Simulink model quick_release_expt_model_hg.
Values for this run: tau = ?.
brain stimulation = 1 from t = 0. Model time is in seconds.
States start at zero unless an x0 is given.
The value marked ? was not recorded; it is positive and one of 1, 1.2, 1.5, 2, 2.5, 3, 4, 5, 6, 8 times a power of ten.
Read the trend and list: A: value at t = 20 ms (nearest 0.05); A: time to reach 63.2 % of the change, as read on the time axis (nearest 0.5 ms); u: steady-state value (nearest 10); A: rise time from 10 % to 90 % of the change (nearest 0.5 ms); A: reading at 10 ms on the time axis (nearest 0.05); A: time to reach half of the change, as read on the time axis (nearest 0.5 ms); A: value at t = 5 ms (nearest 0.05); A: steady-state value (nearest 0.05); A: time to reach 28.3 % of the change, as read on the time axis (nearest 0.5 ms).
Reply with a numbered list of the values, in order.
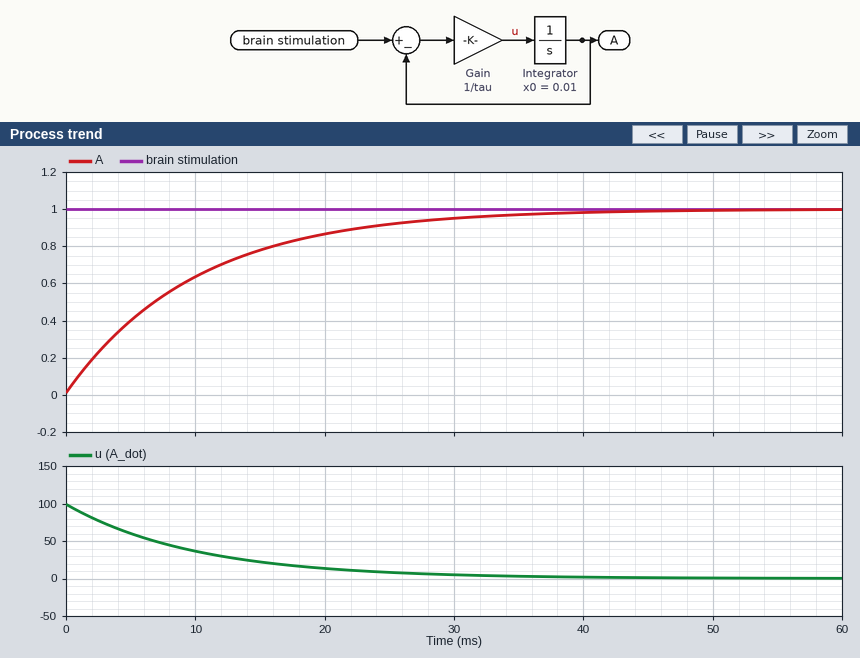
1. 0.85
2. 10.0 ms
3. 0
4. 22.0 ms
5. 0.65
6. 7.0 ms
7. 0.40
8. 1.00
9. 3.5 ms
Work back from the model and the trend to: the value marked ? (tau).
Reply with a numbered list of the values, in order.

1. 0.01
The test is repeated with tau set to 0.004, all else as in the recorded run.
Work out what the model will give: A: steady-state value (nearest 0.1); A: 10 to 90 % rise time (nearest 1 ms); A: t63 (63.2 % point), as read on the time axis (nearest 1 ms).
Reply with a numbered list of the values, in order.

1. 1.0
2. 9 ms
3. 4 ms
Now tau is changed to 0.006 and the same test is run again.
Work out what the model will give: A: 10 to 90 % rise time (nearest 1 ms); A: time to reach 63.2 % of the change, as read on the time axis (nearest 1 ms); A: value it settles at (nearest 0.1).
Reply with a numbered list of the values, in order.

1. 13 ms
2. 6 ms
3. 1.0
